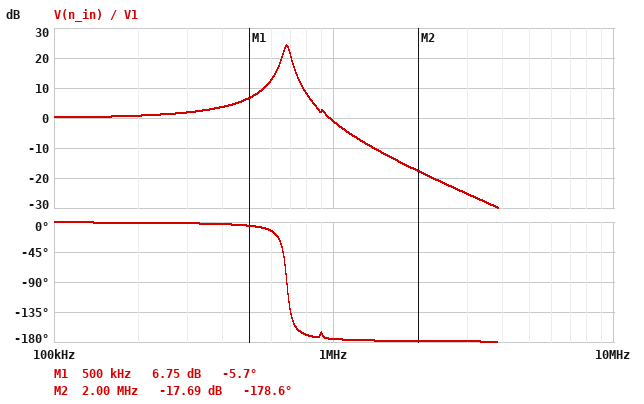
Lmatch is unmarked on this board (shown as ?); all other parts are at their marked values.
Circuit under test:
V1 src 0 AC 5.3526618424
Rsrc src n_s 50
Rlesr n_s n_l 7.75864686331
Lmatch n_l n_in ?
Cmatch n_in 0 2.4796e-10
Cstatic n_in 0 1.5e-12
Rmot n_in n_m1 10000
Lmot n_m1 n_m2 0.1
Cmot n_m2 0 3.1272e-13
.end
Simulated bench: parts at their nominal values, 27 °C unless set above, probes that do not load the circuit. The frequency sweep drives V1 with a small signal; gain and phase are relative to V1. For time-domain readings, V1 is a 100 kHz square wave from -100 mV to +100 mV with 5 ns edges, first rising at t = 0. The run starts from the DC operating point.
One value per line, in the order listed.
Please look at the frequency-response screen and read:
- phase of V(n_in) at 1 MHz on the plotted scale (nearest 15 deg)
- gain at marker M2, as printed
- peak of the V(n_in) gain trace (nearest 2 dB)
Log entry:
-180 deg
-17.69 dB
24 dB
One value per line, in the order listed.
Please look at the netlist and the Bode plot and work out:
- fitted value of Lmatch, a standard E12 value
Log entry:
220 µH
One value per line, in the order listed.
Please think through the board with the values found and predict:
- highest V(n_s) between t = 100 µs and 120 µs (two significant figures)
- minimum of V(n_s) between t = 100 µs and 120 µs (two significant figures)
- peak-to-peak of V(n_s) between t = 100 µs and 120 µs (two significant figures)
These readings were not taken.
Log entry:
110 mV
-110 mV
230 mV
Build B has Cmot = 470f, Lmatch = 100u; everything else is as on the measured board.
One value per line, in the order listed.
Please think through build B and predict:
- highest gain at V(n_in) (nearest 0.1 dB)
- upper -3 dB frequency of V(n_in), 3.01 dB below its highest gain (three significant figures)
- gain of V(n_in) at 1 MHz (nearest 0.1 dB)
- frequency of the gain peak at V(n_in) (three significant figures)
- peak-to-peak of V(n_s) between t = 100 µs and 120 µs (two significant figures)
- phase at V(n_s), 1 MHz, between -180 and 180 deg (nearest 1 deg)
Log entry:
20.8 dB
1.05 MHz
20.7 dB
1.01 MHz
220 mV
-44 deg
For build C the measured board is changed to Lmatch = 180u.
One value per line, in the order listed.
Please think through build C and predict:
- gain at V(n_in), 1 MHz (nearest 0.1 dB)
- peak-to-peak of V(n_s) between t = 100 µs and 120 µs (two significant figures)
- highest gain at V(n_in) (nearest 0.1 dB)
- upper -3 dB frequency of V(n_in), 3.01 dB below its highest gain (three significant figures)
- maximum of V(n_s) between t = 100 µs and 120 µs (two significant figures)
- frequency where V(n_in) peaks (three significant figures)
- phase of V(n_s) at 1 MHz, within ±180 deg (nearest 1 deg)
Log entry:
2.3 dB
220 mV
23.3 dB
774 kHz
110 mV
749 kHz
6 deg
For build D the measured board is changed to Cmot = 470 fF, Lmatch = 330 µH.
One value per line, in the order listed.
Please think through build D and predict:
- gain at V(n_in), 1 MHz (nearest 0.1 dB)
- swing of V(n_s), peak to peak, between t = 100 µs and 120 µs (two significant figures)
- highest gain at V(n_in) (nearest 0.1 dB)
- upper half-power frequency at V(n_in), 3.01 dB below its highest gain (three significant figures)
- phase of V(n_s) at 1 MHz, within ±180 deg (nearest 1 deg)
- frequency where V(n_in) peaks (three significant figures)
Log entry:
-7.0 dB
210 mV
25.9 dB
567 kHz
2 deg
553 kHz
